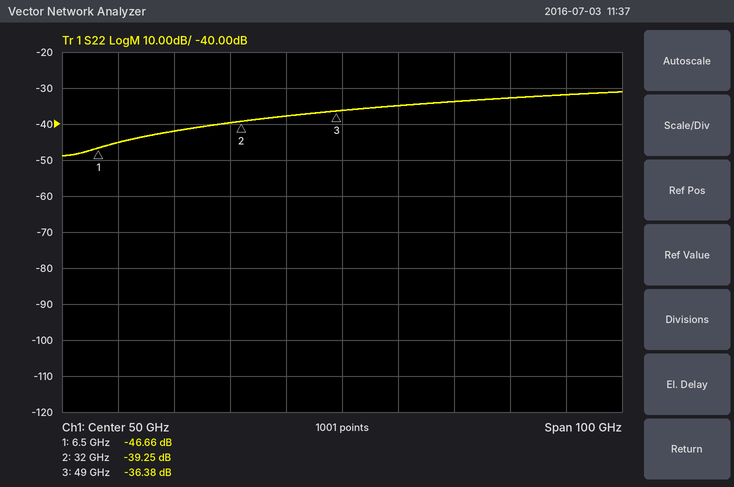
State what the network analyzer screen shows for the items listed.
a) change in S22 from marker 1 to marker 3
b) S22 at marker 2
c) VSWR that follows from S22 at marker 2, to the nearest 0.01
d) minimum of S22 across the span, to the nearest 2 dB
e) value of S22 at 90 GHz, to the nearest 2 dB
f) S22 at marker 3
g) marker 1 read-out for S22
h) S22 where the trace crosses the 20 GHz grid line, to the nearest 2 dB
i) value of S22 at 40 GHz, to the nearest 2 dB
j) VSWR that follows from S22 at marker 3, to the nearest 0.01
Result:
10.28 dB
-39.25 dB
1.02
-48 dB
-32 dB
-36.38 dB
-46.66 dB
-42 dB
-38 dB
1.03
